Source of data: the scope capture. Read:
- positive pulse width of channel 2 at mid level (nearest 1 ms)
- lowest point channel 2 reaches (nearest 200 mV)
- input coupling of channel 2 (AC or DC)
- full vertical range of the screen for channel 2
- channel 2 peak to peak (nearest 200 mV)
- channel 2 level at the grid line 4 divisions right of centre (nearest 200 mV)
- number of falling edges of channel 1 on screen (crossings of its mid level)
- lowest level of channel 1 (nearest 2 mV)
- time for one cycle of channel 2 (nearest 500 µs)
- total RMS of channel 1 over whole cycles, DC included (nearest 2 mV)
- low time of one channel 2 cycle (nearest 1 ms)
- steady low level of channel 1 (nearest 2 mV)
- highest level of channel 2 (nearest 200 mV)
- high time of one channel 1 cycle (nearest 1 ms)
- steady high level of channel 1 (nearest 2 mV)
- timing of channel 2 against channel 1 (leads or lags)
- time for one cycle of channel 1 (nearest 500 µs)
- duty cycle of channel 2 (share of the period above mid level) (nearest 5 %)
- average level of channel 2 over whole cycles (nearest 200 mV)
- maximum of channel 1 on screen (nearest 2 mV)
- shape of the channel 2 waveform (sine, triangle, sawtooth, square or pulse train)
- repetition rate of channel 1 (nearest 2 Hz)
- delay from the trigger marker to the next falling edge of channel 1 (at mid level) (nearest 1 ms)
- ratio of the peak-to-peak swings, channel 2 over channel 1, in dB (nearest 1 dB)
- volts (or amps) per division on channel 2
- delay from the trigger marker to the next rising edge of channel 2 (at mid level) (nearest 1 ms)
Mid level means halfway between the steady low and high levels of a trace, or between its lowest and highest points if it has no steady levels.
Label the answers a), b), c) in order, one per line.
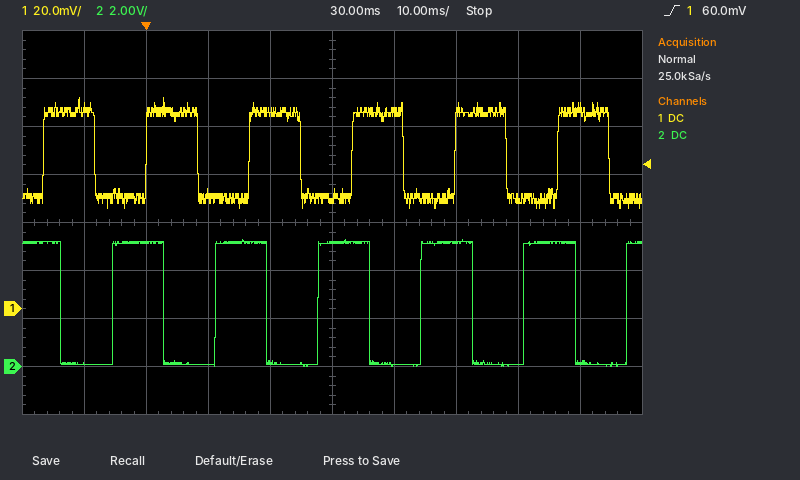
a) 8 ms
b) 0.0 V
c) DC
d) 16 V
e) 5.2 V
f) 200 mV
g) 6
h) 42 mV
i) 16.5 ms
j) 66 mV
k) 8 ms
l) 46 mV
m) 5.2 V
n) 8 ms
o) 82 mV
p) leads
q) 16.5 ms
r) 50 %
s) 2.6 V
t) 88 mV
u) square
v) 60 Hz
w) 8 ms
x) 41 dB
y) 2 V
z) 11 ms
